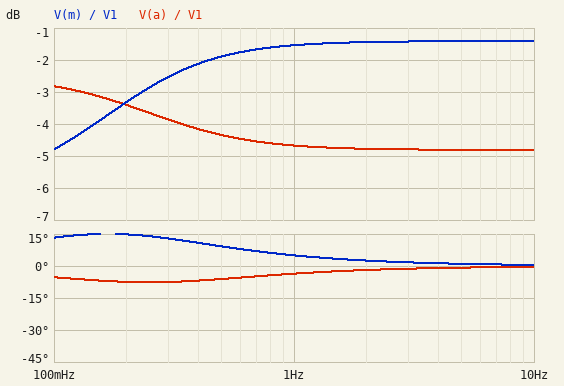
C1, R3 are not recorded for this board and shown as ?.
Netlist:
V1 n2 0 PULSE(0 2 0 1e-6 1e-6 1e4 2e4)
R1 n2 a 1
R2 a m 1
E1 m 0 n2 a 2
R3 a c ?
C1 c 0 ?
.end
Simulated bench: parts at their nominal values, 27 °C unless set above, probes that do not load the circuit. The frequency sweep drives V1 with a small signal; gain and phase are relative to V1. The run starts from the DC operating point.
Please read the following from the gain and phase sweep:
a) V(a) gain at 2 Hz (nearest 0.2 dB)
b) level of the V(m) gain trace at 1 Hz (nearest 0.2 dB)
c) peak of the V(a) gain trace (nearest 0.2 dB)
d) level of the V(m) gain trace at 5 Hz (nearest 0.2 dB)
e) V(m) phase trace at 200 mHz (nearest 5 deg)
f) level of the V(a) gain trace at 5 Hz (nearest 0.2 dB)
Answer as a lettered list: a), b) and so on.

a) -4.8 dB
b) -1.6 dB
c) -2.8 dB
d) -1.4 dB
e) 15 deg
f) -4.8 dB
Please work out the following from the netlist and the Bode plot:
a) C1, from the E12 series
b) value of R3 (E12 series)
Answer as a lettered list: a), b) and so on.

a) 680 mF
b) 0.82 Ω
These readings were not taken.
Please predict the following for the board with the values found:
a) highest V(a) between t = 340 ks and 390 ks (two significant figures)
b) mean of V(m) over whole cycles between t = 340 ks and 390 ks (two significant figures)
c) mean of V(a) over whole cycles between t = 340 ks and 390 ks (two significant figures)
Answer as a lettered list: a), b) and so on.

a) 1.5 V
b) 500 mV
c) 750 mV
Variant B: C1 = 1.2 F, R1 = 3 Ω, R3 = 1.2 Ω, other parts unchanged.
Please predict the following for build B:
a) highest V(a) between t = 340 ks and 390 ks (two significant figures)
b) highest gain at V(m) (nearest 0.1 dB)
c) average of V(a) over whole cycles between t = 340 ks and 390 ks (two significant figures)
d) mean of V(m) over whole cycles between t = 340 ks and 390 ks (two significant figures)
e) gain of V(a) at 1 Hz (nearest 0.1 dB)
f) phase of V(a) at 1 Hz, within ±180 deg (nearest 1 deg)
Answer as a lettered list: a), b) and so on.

a) 1.4 V
b) -1.1 dB
c) 700 mV
d) 600 mV
e) -5.0 dB
f) -1 deg
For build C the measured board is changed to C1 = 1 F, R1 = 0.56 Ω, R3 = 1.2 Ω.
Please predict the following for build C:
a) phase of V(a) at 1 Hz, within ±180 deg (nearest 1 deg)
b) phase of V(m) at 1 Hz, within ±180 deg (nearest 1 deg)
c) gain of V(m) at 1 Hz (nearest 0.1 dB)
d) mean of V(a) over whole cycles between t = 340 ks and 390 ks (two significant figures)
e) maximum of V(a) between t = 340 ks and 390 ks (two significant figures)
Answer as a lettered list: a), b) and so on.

a) -1 deg
b) 2 deg
c) -3.7 dB
d) 790 mV
e) 1.6 V
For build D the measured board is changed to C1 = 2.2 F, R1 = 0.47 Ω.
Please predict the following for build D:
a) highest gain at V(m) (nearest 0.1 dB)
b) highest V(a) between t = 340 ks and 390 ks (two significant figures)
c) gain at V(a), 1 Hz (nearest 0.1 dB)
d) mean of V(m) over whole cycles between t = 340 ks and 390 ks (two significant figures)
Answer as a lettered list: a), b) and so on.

a) -3.1 dB
b) 1.6 V
c) -3.7 dB
d) 390 mV
